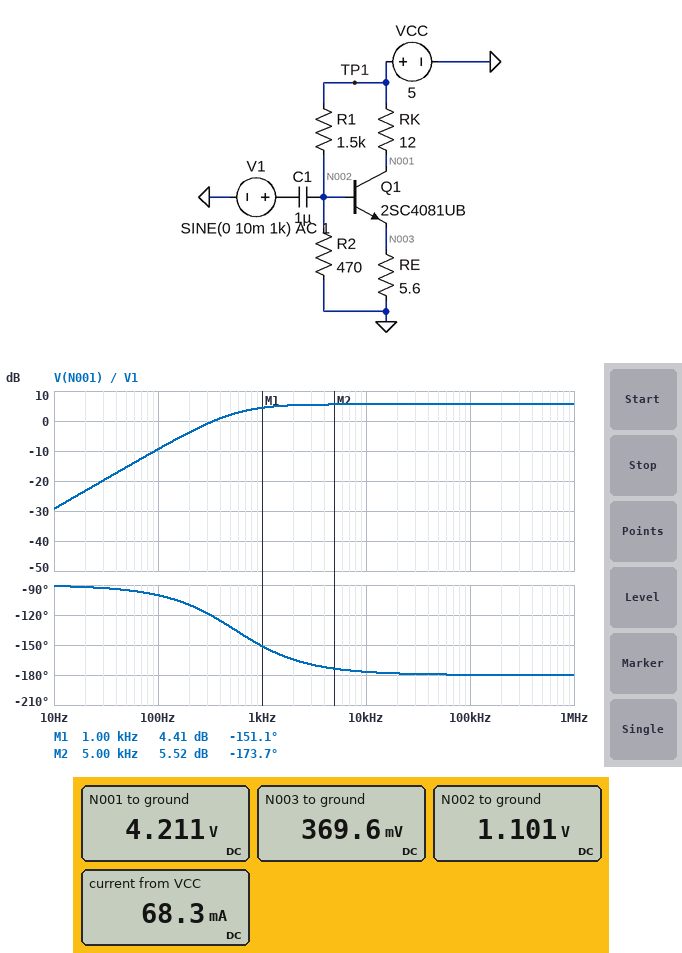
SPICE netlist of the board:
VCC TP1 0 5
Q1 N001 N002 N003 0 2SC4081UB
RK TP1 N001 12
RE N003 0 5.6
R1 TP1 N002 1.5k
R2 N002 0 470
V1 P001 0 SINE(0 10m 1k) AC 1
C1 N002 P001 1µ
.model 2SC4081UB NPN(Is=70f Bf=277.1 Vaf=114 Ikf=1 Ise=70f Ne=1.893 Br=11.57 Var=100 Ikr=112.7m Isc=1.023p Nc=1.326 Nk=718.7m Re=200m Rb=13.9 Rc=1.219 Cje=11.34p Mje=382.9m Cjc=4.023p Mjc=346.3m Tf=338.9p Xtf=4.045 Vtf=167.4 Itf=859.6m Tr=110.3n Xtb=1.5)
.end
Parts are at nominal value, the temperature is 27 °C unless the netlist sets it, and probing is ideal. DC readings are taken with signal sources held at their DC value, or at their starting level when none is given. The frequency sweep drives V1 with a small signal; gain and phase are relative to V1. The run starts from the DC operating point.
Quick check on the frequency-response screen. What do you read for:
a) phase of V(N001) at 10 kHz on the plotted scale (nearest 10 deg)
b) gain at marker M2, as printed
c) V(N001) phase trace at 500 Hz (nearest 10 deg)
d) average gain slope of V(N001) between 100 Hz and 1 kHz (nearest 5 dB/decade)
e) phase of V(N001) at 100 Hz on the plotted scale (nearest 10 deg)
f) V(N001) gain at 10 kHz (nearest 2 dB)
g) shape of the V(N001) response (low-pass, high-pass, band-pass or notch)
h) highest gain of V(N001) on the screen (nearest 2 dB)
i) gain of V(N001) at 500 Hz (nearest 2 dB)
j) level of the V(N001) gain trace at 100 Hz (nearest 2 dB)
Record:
-180 deg
5.52 dB
-130 deg
15 dB/decade
-100 deg
6 dB
high-pass
6 dB
2 dB
-10 dB
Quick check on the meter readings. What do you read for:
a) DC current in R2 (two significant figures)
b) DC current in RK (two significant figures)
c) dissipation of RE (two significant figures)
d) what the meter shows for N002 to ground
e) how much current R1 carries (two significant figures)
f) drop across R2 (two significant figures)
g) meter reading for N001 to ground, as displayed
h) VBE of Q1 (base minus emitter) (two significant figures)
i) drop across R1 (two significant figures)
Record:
2.3 mA
66 mA
24 mW
1.101 V
2.6 mA
1.1 V
4.211 V
730 mV
3.9 V
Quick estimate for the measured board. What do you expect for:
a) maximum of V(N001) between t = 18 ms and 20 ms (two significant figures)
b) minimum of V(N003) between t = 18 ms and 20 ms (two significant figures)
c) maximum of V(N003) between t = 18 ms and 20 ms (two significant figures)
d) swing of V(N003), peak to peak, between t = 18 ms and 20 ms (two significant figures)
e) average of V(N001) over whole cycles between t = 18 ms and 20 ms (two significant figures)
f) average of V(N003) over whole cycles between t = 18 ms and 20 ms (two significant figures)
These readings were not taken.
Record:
4.2 V
360 mV
380 mV
16 mV
4.2 V
370 mV
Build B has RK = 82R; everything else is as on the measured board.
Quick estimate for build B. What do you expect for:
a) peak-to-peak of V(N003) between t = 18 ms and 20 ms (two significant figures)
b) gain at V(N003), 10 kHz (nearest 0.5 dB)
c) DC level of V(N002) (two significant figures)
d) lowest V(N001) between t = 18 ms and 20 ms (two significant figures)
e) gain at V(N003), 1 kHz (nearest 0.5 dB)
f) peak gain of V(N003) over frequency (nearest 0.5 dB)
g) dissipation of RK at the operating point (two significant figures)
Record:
1.5 mV
-9.5 dB
1.0 V
480 mV
-22.5 dB
-8.5 dB
250 mW
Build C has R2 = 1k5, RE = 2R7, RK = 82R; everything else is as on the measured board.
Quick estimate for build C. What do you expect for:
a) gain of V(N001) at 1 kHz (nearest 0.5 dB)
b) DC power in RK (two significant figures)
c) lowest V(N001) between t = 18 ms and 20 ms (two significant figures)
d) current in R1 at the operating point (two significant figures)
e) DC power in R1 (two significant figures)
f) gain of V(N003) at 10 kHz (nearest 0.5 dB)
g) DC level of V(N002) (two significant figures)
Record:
-28.0 dB
270 mW
290 mV
2.7 mA
11 mW
-19.5 dB
920 mV
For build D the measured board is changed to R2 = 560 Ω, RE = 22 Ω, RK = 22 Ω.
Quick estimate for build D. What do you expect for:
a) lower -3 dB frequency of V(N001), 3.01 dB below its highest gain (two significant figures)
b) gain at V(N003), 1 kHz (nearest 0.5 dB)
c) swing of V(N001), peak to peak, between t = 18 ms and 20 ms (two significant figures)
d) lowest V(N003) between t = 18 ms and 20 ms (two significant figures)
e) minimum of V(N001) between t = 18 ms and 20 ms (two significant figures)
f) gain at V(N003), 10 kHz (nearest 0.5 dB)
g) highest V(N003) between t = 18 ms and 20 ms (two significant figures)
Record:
420 Hz
-1.0 dB
17 mV
610 mV
4.4 V
-0.5 dB
630 mV
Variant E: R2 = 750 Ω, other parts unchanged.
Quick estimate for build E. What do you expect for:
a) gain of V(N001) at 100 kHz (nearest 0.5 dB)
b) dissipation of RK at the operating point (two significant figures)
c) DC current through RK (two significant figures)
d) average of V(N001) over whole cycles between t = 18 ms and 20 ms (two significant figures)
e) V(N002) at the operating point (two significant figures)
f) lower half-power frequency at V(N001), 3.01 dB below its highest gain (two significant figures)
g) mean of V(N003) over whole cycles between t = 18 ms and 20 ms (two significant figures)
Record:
6.0 dB
160 mW
120 mA
3.6 V
1.4 V
450 Hz
660 mV
